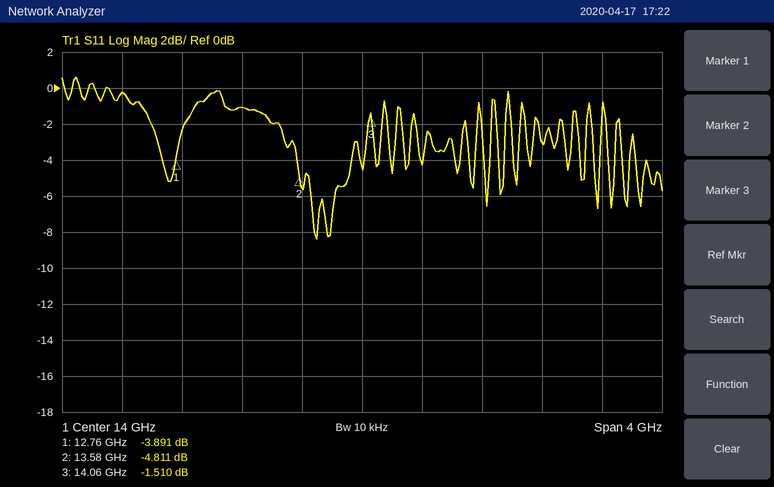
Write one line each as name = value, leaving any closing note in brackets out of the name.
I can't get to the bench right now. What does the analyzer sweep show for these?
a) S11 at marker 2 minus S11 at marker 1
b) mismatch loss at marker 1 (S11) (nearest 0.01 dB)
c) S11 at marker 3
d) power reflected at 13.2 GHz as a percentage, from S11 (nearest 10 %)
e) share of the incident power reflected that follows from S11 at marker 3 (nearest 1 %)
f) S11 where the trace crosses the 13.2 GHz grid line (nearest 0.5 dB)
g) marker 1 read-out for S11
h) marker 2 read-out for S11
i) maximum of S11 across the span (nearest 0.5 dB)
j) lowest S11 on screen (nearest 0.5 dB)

S11 at marker 2 minus S11 at marker 1 = -0.920 dB
mismatch loss at marker 1 (S11) = 2.28 dB
S11 at marker 3 = -1.510 dB
power reflected at 13.2 GHz as a percentage, from S11 = 80 %
share of the incident power reflected that follows from S11 at marker 3 = 71 %
S11 where the trace crosses the 13.2 GHz grid line = -1.0 dB
marker 1 read-out for S11 = -3.891 dB
marker 2 read-out for S11 = -4.811 dB
maximum of S11 across the span = 0.5 dB
lowest S11 on screen = -8.5 dB
